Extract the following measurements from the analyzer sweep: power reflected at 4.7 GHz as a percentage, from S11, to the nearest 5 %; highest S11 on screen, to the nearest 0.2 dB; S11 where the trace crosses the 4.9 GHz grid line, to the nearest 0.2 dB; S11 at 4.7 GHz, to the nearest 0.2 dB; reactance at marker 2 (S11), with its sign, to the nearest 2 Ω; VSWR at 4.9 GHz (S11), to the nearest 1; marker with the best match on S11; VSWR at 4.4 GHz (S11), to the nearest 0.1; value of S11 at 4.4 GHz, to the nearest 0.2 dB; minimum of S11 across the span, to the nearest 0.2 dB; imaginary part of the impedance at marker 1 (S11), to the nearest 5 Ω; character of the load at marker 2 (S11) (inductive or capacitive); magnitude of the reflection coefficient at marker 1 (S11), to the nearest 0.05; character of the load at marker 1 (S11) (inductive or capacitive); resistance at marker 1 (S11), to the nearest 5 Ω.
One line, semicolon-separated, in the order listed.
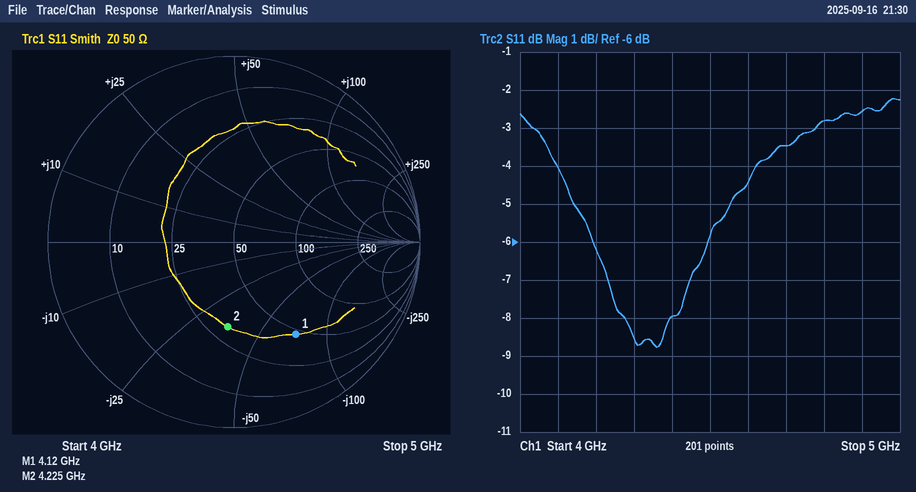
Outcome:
45 %; -2.2 dB; -2.6 dB; -3.4 dB; -36 Ω; 7; marker 2; 2.3; -8.0 dB; -8.8 dB; -70 Ω; capacitive; 0.60; capacitive; 45 Ω
